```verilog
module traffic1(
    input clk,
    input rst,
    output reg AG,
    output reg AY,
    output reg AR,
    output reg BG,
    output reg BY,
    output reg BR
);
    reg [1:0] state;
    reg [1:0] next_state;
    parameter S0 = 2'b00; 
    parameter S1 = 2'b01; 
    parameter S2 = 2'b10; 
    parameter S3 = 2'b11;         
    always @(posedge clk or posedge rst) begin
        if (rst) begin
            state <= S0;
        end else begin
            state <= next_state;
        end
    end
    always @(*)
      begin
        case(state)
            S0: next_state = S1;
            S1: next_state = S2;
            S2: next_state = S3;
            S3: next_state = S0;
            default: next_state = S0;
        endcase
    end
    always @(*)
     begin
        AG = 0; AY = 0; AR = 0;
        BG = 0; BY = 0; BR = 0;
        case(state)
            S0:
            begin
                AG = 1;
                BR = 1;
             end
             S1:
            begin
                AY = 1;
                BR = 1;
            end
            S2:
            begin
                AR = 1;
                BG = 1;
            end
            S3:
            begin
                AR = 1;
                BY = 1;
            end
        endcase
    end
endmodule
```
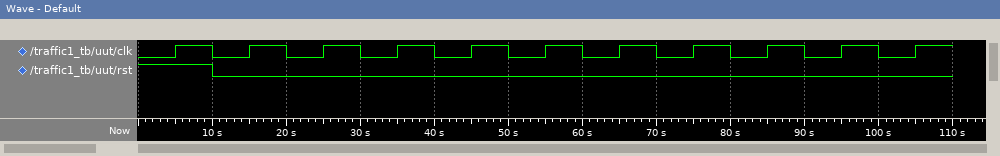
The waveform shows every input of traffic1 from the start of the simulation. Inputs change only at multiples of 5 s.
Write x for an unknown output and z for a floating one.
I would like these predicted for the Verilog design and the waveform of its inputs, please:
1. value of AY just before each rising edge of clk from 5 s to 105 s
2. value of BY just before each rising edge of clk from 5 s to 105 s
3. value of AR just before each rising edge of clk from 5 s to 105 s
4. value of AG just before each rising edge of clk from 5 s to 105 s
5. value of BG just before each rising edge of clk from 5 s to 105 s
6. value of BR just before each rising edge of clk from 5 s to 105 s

0 0 1 0 0 0 1 0 0 0 1
0 0 0 0 1 0 0 0 1 0 0
0 0 0 1 1 0 0 1 1 0 0
1 1 0 0 0 1 0 0 0 1 0
0 0 0 1 0 0 0 1 0 0 0
1 1 1 0 0 1 1 0 0 1 1
